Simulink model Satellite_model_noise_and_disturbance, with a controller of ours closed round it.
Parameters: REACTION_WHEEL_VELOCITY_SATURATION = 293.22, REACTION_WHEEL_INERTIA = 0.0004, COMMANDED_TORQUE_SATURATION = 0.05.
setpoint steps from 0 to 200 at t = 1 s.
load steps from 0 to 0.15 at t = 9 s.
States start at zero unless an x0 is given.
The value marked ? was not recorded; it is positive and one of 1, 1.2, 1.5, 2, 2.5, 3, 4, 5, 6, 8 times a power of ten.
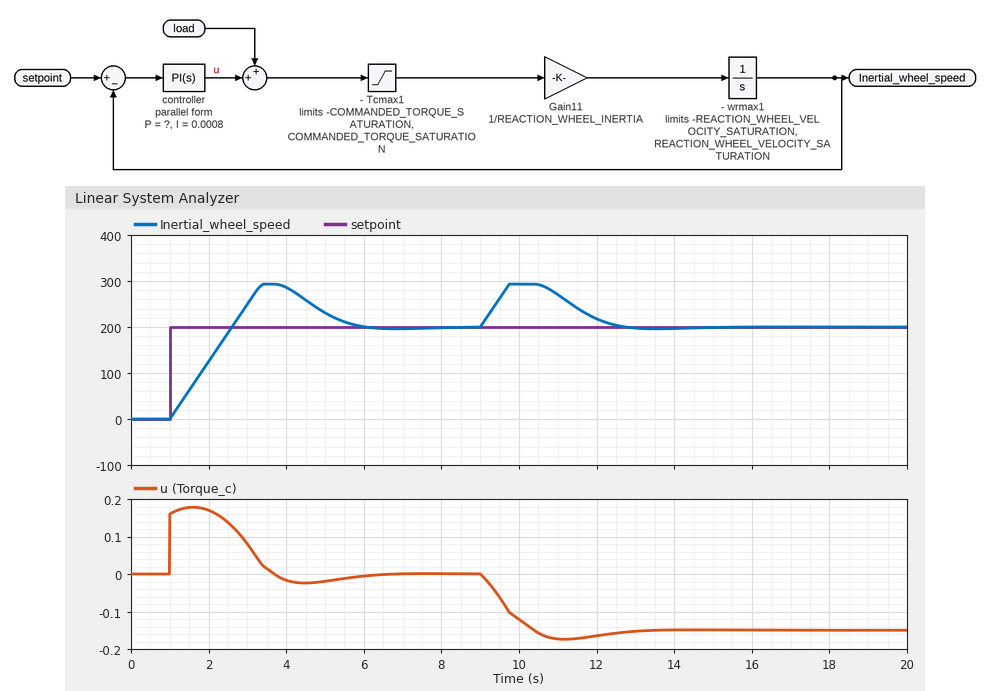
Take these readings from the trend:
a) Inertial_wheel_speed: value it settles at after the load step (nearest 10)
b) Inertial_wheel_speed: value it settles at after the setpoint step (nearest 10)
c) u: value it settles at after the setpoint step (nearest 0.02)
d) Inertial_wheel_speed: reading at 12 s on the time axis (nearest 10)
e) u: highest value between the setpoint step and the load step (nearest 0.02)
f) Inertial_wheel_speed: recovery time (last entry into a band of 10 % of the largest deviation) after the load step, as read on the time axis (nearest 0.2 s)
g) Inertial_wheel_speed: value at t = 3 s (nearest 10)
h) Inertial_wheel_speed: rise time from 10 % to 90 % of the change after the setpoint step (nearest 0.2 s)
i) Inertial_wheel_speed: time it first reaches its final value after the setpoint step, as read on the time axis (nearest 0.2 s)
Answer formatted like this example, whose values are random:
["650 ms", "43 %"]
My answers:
["200", "200", "0.00", "220", "0.18", "12.2 s", "250", "1.2 s", "2.6 s"]
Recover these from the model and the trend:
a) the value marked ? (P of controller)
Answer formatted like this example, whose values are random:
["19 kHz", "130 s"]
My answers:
["0.0008"]
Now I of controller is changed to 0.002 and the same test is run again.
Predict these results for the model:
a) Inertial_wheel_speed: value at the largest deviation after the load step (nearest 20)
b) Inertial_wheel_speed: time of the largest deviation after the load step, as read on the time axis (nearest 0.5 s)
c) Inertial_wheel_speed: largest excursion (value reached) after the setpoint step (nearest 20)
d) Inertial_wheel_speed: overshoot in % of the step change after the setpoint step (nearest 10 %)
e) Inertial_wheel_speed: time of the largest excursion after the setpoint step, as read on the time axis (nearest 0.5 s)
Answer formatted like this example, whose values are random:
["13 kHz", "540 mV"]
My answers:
["280", "10.0 s", "300", "50 %", "3.5 s"]
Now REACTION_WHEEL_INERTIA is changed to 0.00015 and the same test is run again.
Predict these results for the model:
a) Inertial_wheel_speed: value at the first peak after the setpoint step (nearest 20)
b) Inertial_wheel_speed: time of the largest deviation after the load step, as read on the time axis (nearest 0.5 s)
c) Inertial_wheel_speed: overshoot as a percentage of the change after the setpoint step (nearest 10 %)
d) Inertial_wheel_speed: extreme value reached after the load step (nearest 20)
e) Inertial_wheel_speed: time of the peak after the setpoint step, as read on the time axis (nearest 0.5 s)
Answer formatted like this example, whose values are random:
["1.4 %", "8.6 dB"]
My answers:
["240", "9.5 s", "20 %", "300", "2.0 s"]
